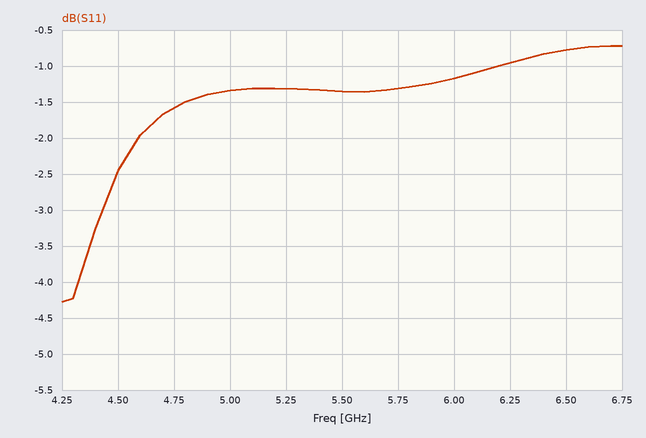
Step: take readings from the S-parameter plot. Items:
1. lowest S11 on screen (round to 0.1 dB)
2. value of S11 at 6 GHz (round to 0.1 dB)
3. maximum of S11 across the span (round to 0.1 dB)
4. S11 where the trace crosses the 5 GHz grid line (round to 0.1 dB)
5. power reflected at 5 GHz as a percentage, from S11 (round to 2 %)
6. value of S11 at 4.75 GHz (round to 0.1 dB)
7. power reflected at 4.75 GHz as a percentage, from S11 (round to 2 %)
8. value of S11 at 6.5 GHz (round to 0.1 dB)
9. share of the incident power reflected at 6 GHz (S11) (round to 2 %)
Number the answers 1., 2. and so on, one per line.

1. -4.3 dB
2. -1.2 dB
3. -0.7 dB
4. -1.3 dB
5. 74 %
6. -1.6 dB
7. 70 %
8. -0.8 dB
9. 76 %
